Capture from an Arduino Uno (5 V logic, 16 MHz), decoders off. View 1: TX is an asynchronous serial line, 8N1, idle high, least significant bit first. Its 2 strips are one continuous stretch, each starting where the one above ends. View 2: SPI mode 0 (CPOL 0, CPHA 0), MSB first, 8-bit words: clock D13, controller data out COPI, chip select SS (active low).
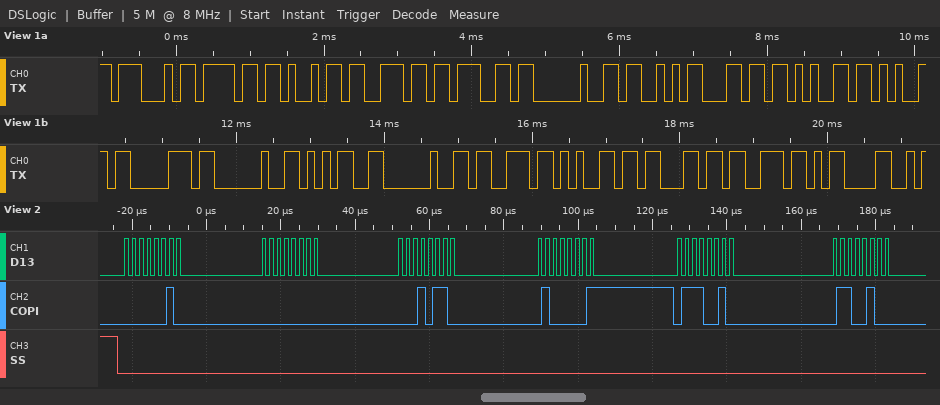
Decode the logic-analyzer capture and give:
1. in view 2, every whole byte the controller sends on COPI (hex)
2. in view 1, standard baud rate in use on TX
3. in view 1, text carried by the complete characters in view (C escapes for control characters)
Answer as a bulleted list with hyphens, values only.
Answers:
- 02 00 16 41 72 64
- 9600 baud
- "Going Sleep 5 secs\r"
